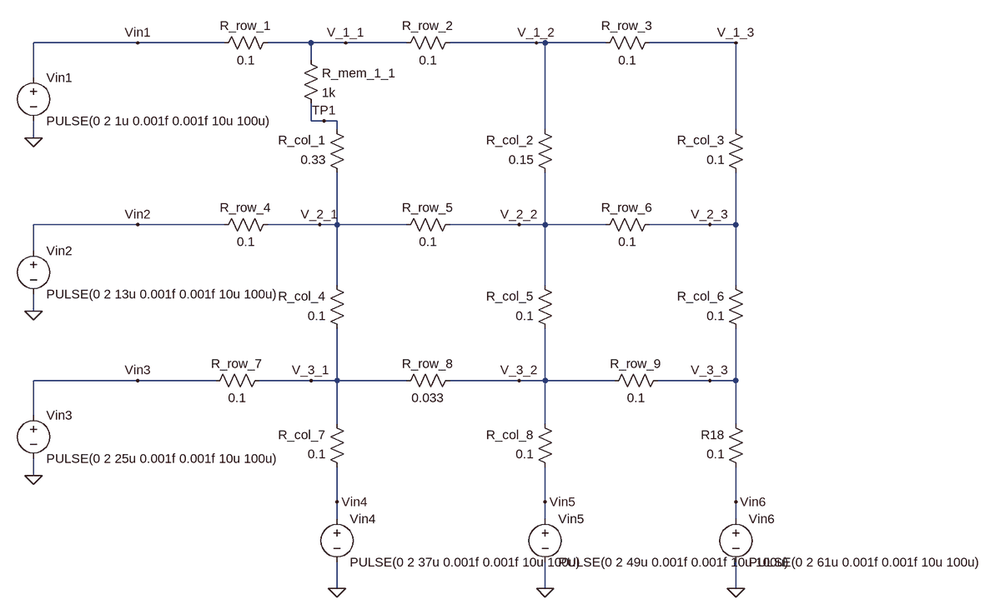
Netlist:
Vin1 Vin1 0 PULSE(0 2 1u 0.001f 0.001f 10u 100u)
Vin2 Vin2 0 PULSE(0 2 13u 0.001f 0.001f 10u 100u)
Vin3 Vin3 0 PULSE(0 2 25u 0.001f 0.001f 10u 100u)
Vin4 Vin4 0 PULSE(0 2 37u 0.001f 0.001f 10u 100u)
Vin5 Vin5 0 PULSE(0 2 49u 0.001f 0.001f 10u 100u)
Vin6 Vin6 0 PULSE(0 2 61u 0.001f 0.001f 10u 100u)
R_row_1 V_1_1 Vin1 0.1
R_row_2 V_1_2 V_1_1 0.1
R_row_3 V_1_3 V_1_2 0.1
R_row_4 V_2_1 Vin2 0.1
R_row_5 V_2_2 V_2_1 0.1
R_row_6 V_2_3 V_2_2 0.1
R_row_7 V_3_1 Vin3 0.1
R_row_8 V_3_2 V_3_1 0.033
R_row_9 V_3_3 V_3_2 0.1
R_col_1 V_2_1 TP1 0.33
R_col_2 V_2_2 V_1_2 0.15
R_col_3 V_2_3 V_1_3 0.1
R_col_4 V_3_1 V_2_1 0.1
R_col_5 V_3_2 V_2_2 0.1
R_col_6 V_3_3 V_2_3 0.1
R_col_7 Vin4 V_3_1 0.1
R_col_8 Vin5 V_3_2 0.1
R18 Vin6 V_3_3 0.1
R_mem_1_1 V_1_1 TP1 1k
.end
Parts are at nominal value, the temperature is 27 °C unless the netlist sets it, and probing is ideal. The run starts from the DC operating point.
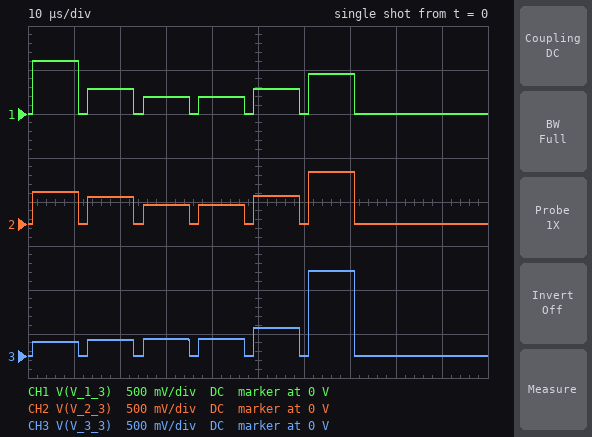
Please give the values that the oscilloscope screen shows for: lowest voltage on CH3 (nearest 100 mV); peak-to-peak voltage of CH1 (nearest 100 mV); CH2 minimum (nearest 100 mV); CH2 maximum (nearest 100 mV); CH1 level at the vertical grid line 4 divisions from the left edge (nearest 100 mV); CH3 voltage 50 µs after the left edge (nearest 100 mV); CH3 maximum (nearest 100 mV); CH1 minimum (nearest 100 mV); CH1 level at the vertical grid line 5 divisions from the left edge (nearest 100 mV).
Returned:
0 V
600 mV
0 V
600 mV
200 mV
300 mV
1.0 V
0 V
300 mV
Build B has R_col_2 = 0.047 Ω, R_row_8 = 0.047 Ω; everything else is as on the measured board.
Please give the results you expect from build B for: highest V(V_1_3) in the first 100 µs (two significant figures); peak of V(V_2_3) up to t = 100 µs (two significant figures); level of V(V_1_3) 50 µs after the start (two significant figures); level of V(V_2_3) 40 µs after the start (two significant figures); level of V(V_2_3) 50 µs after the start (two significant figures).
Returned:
500 mV
600 mV
320 mV
200 mV
340 mV
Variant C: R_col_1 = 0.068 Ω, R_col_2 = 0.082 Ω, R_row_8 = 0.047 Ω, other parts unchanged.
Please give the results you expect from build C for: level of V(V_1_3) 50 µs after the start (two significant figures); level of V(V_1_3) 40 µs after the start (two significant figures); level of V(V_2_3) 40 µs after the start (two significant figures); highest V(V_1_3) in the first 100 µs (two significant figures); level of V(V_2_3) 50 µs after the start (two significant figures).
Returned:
310 mV
190 mV
200 mV
550 mV
340 mV
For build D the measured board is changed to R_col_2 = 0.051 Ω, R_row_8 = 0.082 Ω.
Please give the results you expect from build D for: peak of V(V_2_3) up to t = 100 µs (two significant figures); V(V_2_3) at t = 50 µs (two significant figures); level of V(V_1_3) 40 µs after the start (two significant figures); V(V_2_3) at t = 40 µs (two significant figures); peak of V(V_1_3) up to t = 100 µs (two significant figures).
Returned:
620 mV
370 mV
170 mV
180 mV
510 mV
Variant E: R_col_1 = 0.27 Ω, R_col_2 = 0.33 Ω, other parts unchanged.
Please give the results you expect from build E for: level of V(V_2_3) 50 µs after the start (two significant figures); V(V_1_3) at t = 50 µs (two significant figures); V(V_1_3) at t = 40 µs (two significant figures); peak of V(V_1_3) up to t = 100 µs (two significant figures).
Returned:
320 mV
270 mV
180 mV
660 mV
